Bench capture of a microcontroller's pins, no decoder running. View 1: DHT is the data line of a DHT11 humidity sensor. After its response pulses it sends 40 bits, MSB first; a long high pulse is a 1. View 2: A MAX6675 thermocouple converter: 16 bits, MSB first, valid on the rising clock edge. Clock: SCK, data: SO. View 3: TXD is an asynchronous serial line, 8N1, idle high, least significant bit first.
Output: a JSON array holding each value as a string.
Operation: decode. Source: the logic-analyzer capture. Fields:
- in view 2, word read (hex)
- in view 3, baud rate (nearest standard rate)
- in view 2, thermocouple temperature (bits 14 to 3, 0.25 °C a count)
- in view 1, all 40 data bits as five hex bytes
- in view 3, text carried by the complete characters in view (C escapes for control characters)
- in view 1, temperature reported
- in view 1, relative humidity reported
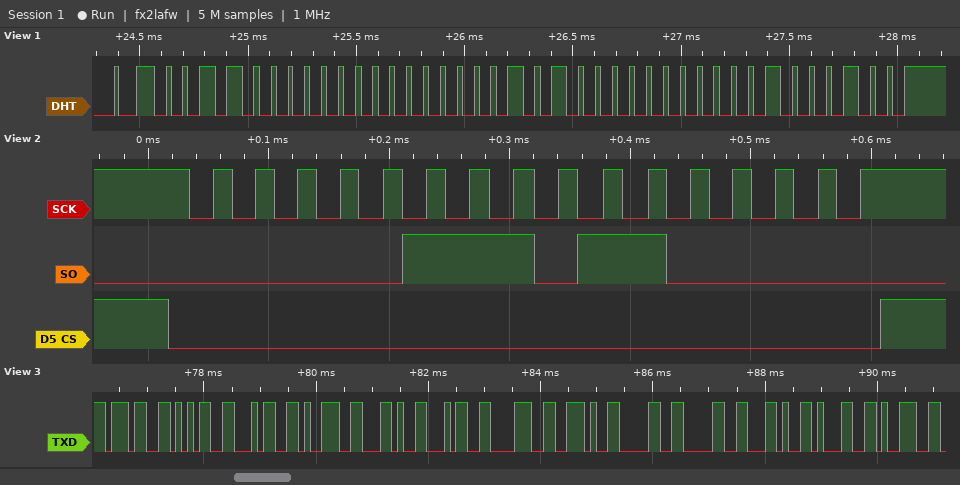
["0x0760", "9600 baud", "59.00 °C", "30 00 14 00 44", "\"7549,48.00,19\"", "20.0 °C", "48 %"]
